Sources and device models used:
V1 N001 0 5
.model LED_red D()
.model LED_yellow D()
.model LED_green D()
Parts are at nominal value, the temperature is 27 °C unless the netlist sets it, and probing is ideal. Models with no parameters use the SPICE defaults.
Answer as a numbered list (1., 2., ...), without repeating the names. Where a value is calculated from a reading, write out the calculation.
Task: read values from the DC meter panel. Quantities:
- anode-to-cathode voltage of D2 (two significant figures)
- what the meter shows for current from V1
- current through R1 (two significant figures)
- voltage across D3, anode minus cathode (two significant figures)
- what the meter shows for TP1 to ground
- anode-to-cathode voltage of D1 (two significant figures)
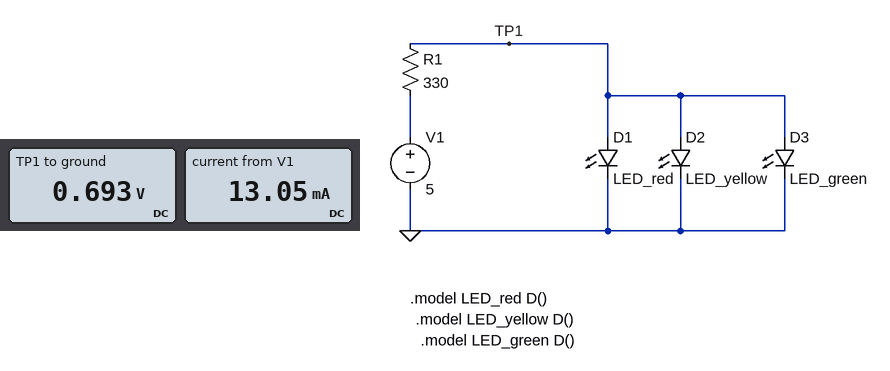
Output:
1. 693 mV = 690 mV
2. 13.05 mA
3. (5 V - 693 mV) / 330 Ω = 13 mA
4. 693 mV = 690 mV
5. 0.693 V
6. 693 mV = 690 mV
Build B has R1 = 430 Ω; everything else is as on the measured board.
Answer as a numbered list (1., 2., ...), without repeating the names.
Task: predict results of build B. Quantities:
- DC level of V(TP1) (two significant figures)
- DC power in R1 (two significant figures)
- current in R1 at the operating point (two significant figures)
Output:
1. 690 mV
2. 43 mW
3. 10 mA
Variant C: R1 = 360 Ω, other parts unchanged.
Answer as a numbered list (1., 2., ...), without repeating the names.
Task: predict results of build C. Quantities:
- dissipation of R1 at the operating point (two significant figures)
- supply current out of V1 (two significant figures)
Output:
1. 52 mW
2. 12 mA
